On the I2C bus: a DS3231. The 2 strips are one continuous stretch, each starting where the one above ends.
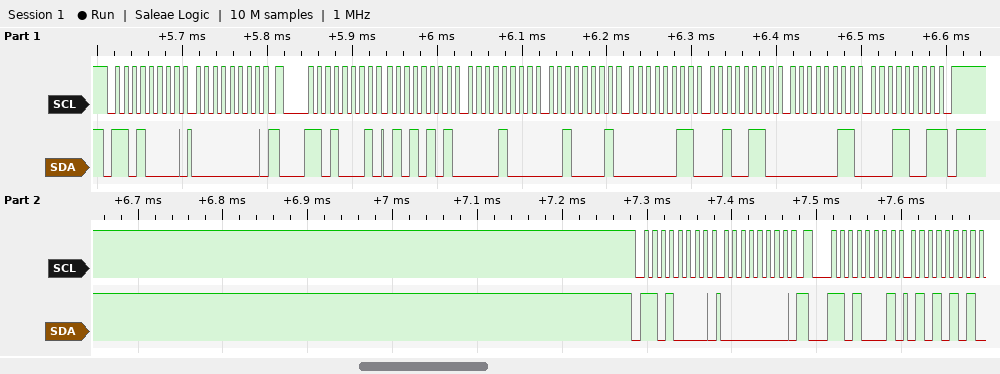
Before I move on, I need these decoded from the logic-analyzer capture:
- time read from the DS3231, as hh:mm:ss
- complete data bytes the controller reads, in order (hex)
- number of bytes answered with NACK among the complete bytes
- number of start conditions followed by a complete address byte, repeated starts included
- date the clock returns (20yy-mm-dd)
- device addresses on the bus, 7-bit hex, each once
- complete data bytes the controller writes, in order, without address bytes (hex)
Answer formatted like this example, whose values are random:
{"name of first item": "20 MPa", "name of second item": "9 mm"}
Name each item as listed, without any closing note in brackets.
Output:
{"time read from the DS3231, as hh:mm:ss": "21:08:55", "complete data bytes the controller reads, in order": "55 08 21 03 26 03 19 55", "number of bytes answered with NACK among the complete bytes": "1", "number of start conditions followed by a complete address byte, repeated starts included": "4", "date the clock returns": "2019-03-26", "device addresses on the bus, 7-bit hex, each once": "0x68", "complete data bytes the controller writes, in order, without address bytes": "00 00"}
